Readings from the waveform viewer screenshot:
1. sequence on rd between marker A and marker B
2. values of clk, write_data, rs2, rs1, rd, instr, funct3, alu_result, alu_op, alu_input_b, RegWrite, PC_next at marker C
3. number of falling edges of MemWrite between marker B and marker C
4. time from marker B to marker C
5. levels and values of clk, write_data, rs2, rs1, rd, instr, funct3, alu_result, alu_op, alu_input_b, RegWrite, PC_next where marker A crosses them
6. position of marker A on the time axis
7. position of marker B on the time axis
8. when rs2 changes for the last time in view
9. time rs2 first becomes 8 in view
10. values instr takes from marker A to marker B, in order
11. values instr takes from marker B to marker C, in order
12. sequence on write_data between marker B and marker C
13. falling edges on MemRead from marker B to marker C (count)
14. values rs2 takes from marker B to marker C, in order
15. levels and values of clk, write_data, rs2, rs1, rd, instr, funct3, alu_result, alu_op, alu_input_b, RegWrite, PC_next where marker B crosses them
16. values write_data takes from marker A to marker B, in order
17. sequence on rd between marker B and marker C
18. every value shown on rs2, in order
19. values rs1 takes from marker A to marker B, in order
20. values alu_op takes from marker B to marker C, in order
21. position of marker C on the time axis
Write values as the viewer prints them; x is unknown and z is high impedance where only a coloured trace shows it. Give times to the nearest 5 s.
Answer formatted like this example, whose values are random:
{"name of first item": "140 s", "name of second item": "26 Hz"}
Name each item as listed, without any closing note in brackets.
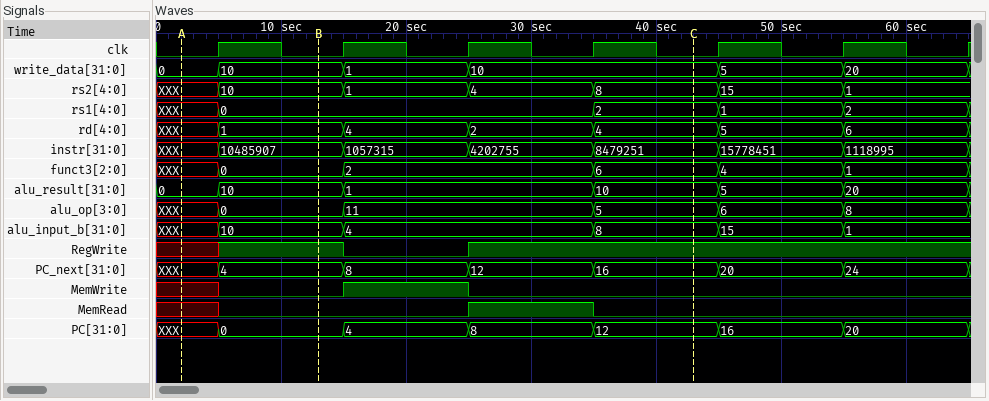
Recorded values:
{"sequence on rd between marker A and marker B": "XXX, 1", "values of clk, write_data, rs2, rs1, rd, instr, funct3, alu_result, alu_op, alu_input_b, RegWrite, PC_next at marker C": "clk=0, write_data=10, rs2=8, rs1=2, rd=4, instr=8479251, funct3=6, alu_result=10, alu_op=5, alu_input_b=8, RegWrite=1, PC_next=16", "number of falling edges of MemWrite between marker B and marker C": "1", "time from marker B to marker C": "30 s", "levels and values of clk, write_data, rs2, rs1, rd, instr, funct3, alu_result, alu_op, alu_input_b, RegWrite, PC_next where marker A crosses them": "clk=0, write_data=0, rs2=XXX, rs1=XXX, rd=XXX, instr=XXX, funct3=XXX, alu_result=0, alu_op=XXX, alu_input_b=XXX, RegWrite=x, PC_next=XXX", "position of marker A on the time axis": "0 s", "position of marker B on the time axis": "15 s", "when rs2 changes for the last time in view": "55 s", "time rs2 first becomes 8 in view": "35 s", "values instr takes from marker A to marker B, in order": "XXX, 10485907", "values instr takes from marker B to marker C, in order": "10485907, 1057315, 4202755, 8479251", "sequence on write_data between marker B and marker C": "10, 1, 10", "falling edges on MemRead from marker B to marker C": "1", "values rs2 takes from marker B to marker C, in order": "10, 1, 4, 8", "levels and values of clk, write_data, rs2, rs1, rd, instr, funct3, alu_result, alu_op, alu_input_b, RegWrite, PC_next where marker B crosses them": "clk=0, write_data=10, rs2=10, rs1=0, rd=1, instr=10485907, funct3=0, alu_result=10, alu_op=0, alu_input_b=10, RegWrite=1, PC_next=4", "values write_data takes from marker A to marker B, in order": "0, 10", "sequence on rd between marker B and marker C": "1, 4, 2, 4", "every value shown on rs2, in order": "XXX, 10, 1, 4, 8, 15, 1", "values rs1 takes from marker A to marker B, in order": "XXX, 0", "values alu_op takes from marker B to marker C, in order": "0, 11, 5", "position of marker C on the time axis": "45 s"}
